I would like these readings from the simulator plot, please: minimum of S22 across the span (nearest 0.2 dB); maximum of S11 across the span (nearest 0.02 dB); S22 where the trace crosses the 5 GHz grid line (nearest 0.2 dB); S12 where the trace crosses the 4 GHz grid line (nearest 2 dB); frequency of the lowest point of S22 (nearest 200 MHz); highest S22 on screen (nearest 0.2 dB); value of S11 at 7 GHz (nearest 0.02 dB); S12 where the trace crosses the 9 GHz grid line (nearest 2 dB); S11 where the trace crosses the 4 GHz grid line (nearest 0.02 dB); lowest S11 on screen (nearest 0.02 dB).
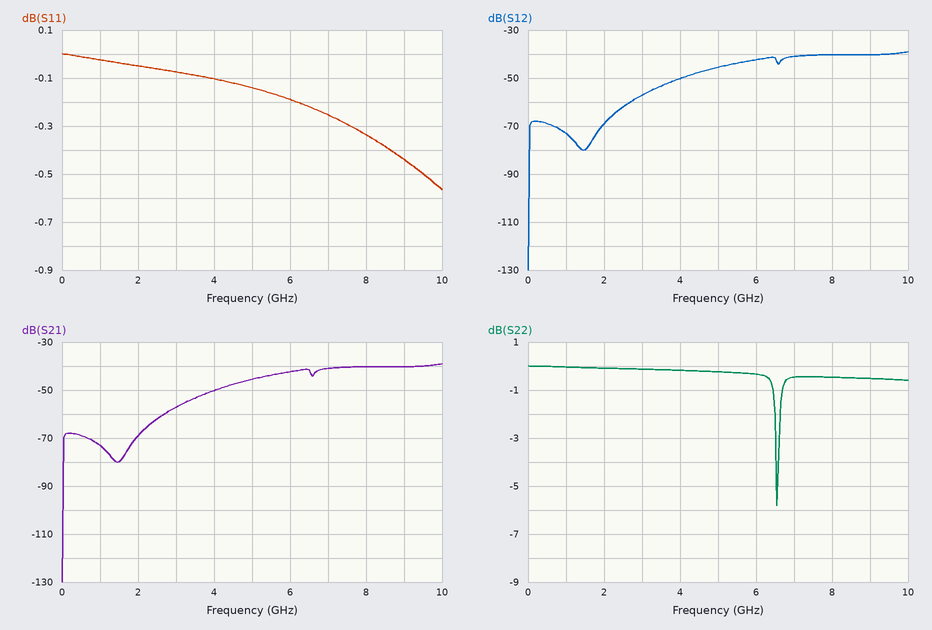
-5.8 dB
0.00 dB
-0.2 dB
-50 dB
6.6 GHz
0.0 dB
-0.26 dB
-40 dB
-0.10 dB
-0.56 dB
